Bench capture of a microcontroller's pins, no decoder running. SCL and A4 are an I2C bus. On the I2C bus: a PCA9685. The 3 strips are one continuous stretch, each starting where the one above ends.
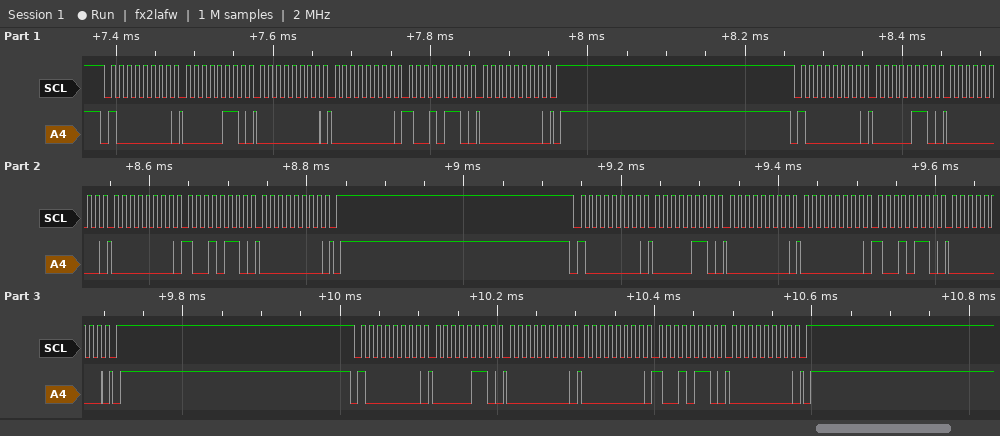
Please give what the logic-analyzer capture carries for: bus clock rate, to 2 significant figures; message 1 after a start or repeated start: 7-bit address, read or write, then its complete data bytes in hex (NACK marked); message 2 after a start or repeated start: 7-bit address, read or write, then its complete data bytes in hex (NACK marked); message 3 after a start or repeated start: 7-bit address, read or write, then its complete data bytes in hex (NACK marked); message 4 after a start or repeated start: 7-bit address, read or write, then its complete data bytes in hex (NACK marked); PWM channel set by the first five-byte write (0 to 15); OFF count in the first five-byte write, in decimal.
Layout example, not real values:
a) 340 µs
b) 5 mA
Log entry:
a) 100 kHz
b) 0x40 write: 06 00 00 96 00
c) 0x40 write: 06 00 00 96 00
d) 0x40 write: 06 00 00 96 00
e) 0x40 write: 06 00 00 96 00
f) 0
g) 150
